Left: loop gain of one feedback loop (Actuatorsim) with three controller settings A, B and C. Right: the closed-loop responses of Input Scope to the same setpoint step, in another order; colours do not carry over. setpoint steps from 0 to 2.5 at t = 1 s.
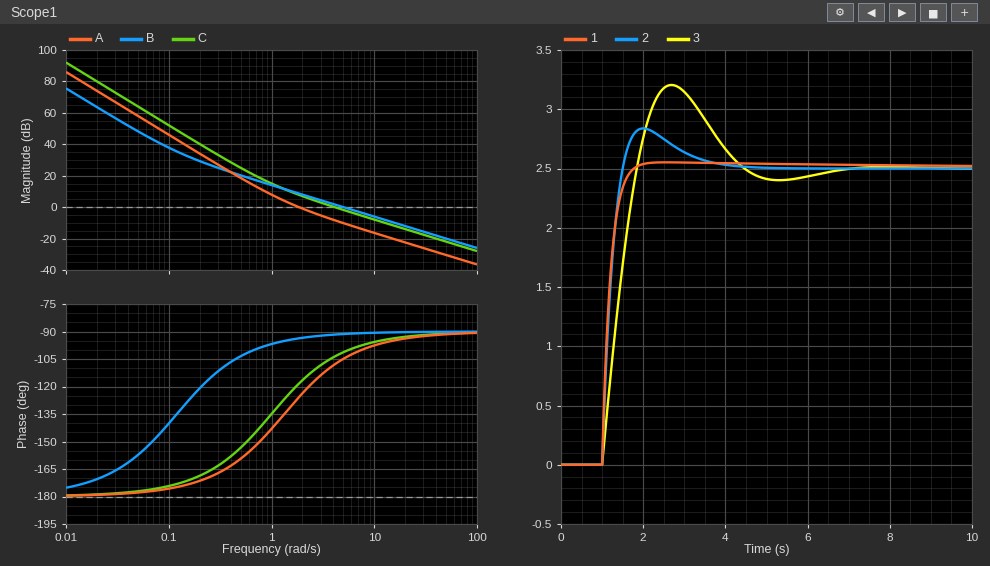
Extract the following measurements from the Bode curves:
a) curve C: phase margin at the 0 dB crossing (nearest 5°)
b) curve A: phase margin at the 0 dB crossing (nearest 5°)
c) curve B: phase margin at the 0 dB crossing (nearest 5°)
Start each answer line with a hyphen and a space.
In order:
- 75°
- 55°
- 90°
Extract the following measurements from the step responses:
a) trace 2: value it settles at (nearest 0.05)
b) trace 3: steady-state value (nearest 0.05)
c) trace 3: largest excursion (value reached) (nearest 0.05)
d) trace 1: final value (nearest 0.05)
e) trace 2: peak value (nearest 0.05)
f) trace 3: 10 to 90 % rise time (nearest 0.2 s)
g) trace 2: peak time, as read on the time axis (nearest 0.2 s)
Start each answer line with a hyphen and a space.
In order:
- 2.50
- 2.50
- 3.20
- 2.50
- 2.85
- 0.6 s
- 2.0 s
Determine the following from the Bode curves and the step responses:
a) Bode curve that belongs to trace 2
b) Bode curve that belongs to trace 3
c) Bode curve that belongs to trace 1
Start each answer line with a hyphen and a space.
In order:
- C
- A
- B
